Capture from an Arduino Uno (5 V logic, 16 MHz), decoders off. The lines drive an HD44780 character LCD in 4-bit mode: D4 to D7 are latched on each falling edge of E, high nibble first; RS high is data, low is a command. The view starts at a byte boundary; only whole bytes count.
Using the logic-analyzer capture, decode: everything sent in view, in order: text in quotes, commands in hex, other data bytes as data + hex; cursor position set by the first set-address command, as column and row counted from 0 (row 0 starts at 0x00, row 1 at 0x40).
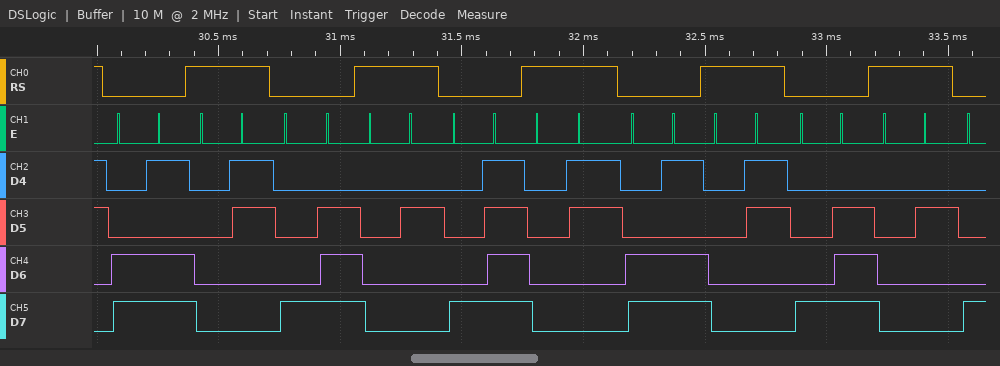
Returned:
0xCD data 03 0x8E data 02 0x8F data 03 0xCD data 03 0x8E data 02
column 13, row 1
